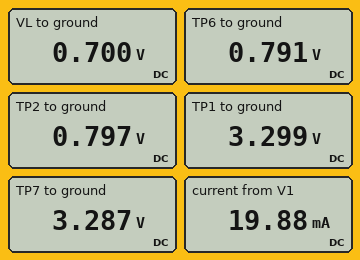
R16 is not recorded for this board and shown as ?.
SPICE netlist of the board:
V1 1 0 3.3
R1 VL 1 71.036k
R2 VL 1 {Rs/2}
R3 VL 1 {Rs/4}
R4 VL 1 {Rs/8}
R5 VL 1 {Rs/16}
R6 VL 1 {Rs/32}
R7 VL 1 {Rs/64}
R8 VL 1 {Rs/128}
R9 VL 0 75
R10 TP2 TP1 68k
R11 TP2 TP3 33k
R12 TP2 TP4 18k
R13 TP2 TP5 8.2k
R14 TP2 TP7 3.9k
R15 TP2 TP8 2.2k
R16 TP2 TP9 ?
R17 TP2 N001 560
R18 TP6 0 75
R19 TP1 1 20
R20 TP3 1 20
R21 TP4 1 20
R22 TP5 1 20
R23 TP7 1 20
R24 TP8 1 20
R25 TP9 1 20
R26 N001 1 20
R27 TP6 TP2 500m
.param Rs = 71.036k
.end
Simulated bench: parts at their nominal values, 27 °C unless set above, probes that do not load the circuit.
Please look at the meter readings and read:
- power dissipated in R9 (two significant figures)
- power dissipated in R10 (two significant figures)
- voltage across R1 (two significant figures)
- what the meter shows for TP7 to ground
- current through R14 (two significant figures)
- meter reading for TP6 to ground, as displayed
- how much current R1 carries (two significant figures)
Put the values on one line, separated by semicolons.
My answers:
6.5 mW; 92 µW; 2.6 V; 3.287 V; 640 µA; 0.791 V; 37 µA
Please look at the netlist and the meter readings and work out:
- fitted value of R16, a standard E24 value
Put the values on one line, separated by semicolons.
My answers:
620 Ω
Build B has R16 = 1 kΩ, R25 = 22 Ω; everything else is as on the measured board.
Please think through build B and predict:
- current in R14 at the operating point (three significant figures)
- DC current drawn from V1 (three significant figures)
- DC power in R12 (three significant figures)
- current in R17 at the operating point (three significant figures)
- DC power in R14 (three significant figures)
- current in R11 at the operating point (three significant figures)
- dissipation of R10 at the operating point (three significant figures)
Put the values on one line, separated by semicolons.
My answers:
661 µA; 18.7 mA; 372 µW; 4.47 mA; 1.70 mW; 78.4 µA; 98.6 µW
